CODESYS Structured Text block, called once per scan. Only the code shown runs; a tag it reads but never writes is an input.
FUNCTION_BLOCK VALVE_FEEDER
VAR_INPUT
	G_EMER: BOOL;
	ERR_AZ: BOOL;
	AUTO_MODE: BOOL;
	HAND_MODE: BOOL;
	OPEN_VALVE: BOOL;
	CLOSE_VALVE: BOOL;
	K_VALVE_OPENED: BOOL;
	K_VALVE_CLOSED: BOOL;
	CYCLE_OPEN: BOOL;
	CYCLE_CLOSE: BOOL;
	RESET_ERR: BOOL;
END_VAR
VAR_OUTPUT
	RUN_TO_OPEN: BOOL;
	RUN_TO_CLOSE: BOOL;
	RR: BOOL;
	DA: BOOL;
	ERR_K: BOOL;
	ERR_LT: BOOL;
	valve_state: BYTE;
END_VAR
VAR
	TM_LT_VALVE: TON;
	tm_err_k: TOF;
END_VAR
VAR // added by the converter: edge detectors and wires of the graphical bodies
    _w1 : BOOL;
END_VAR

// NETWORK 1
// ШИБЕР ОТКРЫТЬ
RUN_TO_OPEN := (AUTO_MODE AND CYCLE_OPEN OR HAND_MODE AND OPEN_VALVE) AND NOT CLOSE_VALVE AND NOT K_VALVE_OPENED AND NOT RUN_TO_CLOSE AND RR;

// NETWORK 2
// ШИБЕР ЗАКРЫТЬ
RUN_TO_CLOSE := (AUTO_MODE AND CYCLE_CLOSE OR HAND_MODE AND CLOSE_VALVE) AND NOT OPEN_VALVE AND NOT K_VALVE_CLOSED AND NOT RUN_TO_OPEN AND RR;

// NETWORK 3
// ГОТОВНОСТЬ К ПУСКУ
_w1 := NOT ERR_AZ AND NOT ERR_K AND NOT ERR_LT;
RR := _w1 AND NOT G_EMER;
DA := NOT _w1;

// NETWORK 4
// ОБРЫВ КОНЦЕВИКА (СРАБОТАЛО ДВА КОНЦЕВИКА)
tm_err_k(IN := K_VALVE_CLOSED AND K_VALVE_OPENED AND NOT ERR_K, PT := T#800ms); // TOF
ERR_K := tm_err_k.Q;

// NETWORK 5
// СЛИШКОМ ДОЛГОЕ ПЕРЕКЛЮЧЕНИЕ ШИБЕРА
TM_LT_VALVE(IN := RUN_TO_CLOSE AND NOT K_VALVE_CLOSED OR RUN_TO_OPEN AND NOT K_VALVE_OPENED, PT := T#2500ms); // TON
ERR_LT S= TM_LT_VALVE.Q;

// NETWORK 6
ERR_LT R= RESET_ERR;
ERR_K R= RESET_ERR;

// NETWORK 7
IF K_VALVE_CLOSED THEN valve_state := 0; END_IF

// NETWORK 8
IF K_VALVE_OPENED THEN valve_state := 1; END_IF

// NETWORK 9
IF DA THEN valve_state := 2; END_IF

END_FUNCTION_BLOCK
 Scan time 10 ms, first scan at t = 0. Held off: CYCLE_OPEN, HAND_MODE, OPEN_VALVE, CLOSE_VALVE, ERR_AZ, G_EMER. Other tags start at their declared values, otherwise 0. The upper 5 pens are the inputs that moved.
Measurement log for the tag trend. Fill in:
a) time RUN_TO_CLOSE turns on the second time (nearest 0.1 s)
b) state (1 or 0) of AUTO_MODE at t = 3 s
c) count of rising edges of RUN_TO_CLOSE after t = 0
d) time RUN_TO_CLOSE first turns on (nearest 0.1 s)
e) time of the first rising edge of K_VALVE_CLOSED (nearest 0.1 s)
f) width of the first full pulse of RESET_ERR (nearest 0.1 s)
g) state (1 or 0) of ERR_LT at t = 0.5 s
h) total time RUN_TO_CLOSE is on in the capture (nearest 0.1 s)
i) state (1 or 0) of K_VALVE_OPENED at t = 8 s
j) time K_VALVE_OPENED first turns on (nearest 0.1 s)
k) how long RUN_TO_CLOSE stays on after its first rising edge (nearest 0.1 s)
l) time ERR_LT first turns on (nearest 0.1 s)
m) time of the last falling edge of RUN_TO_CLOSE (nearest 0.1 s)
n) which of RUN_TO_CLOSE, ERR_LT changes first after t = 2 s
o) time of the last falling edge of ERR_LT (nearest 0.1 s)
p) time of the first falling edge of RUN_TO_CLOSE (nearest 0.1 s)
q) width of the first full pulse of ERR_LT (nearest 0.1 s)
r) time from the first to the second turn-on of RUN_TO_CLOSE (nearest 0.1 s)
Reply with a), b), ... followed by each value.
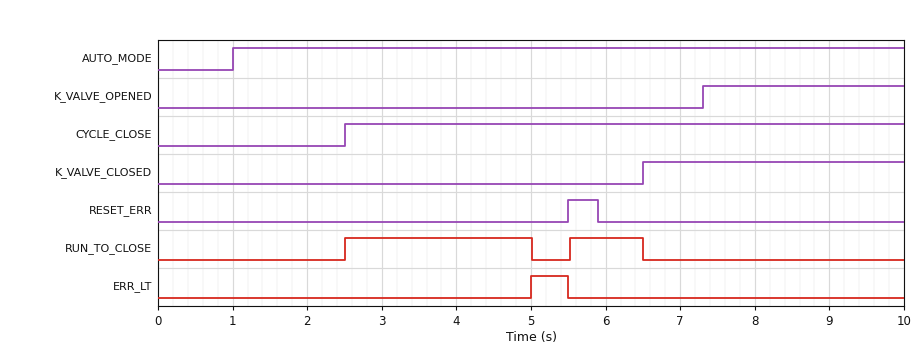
a) 5.5 s
b) 1
c) 2
d) 2.5 s
e) 6.5 s
f) 0.4 s
g) 0
h) 3.5 s
i) 1
j) 7.3 s
k) 2.5 s
l) 5.0 s
m) 6.5 s
n) RUN_TO_CLOSE
o) 5.5 s
p) 5.0 s
q) 0.5 s
r) 3.0 s
